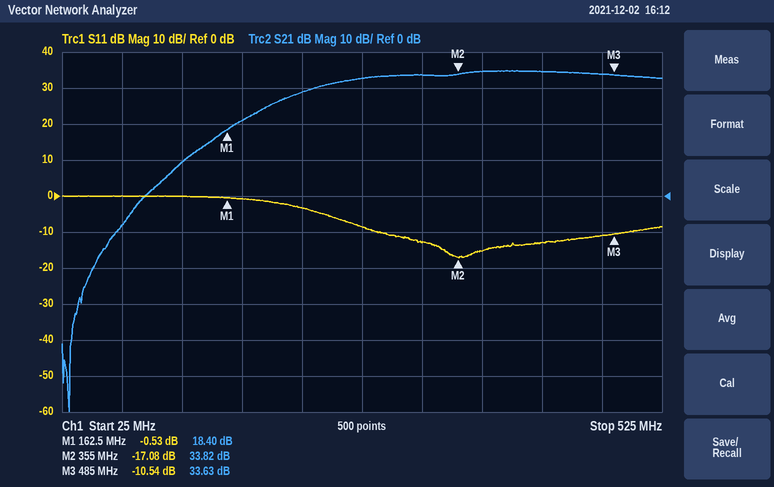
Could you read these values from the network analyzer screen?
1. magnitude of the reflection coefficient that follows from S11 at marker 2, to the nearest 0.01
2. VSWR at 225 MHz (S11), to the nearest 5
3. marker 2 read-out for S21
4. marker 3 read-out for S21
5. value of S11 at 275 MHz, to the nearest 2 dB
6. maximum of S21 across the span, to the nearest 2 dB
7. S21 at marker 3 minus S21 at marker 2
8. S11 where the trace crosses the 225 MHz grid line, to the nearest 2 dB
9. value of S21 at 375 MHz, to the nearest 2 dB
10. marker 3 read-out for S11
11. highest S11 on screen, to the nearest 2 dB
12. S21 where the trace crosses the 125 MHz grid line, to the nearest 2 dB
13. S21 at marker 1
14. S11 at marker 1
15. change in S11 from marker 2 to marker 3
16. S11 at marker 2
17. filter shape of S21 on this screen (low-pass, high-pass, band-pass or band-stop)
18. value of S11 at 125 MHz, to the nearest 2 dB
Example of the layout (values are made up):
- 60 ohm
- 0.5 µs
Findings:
- 0.14
- 5
- 33.82 dB
- 33.63 dB
- -8 dB
- 34 dB
- -0.19 dB
- -4 dB
- 34 dB
- -10.54 dB
- 0 dB
- 10 dB
- 18.40 dB
- -0.53 dB
- 6.54 dB
- -17.08 dB
- high-pass
- 0 dB
